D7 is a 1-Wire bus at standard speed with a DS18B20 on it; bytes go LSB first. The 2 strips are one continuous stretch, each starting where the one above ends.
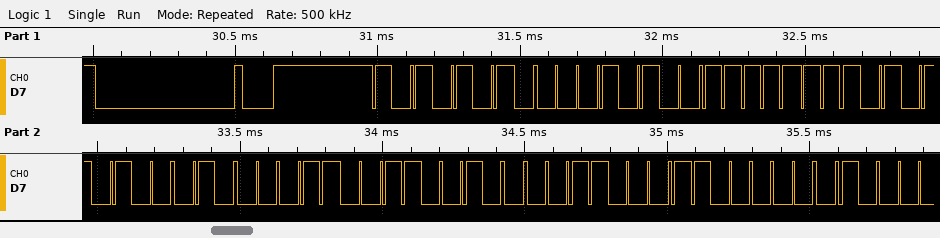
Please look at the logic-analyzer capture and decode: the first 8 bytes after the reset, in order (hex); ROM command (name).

55 28 FF 2A C2 4C 18 03
Match ROM
